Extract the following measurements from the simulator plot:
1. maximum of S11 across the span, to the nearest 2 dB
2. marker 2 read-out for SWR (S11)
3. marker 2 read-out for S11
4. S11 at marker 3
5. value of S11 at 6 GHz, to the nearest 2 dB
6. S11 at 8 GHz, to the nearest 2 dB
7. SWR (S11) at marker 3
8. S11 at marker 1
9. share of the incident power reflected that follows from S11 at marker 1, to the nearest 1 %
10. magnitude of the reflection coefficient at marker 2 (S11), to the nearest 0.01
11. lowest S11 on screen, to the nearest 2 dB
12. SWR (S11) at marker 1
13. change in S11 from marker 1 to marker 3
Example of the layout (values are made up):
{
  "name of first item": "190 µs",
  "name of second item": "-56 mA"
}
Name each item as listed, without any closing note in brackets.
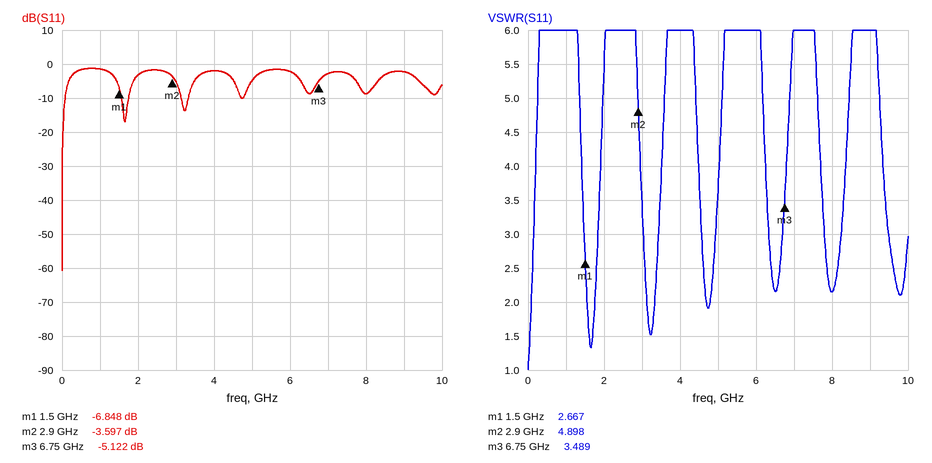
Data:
{
  "maximum of S11 across the span, to the nearest 2 dB": "-2 dB",
  "marker 2 read-out for SWR": "4.898",
  "marker 2 read-out for S11": "-3.597 dB",
  "S11 at marker 3": "-5.122 dB",
  "value of S11 at 6 GHz, to the nearest 2 dB": "-2 dB",
  "S11 at 8 GHz, to the nearest 2 dB": "-8 dB",
  "SWR (S11) at marker 3": "3.489",
  "S11 at marker 1": "-6.848 dB",
  "share of the incident power reflected that follows from S11 at marker 1, to the nearest 1 %": "21 %",
  "magnitude of the reflection coefficient at marker 2 (S11), to the nearest 0.01": "0.66",
  "lowest S11 on screen, to the nearest 2 dB": "-60 dB",
  "SWR (S11) at marker 1": "2.667",
  "change in S11 from marker 1 to marker 3": "1.726 dB"
}
